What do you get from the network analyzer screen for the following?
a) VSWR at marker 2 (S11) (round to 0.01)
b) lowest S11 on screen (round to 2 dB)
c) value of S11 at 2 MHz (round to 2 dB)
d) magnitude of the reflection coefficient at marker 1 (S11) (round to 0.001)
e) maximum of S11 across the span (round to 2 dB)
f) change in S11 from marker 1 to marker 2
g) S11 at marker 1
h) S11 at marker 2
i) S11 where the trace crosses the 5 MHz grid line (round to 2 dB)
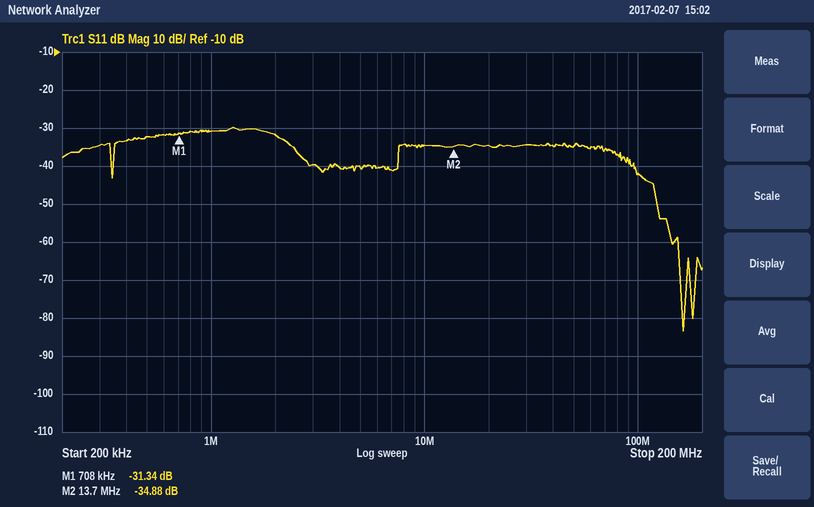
1.04
-84 dB
-32 dB
0.027
-30 dB
-3.54 dB
-31.34 dB
-34.88 dB
-40 dB
